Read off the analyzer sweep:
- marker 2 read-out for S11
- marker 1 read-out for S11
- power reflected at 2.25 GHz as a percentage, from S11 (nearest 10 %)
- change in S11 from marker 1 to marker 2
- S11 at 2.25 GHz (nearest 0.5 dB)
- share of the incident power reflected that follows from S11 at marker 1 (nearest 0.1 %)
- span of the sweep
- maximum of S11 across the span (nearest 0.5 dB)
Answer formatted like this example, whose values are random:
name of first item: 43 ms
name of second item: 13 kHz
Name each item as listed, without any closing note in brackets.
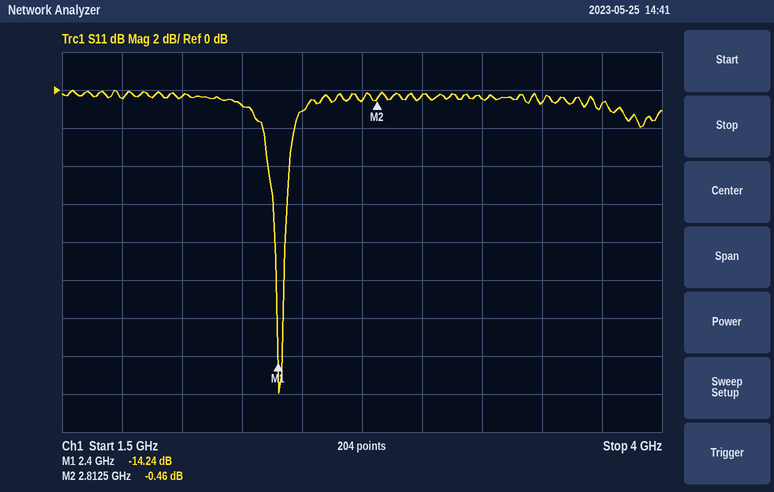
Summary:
marker 2 read-out for S11: -0.46 dB
marker 1 read-out for S11: -14.24 dB
power reflected at 2.25 GHz as a percentage, from S11: 80 %
change in S11 from marker 1 to marker 2: 13.78 dB
S11 at 2.25 GHz: -1.0 dB
share of the incident power reflected that follows from S11 at marker 1: 3.8 %
span of the sweep: 2.5 GHz
maximum of S11 across the span: 0.0 dB
